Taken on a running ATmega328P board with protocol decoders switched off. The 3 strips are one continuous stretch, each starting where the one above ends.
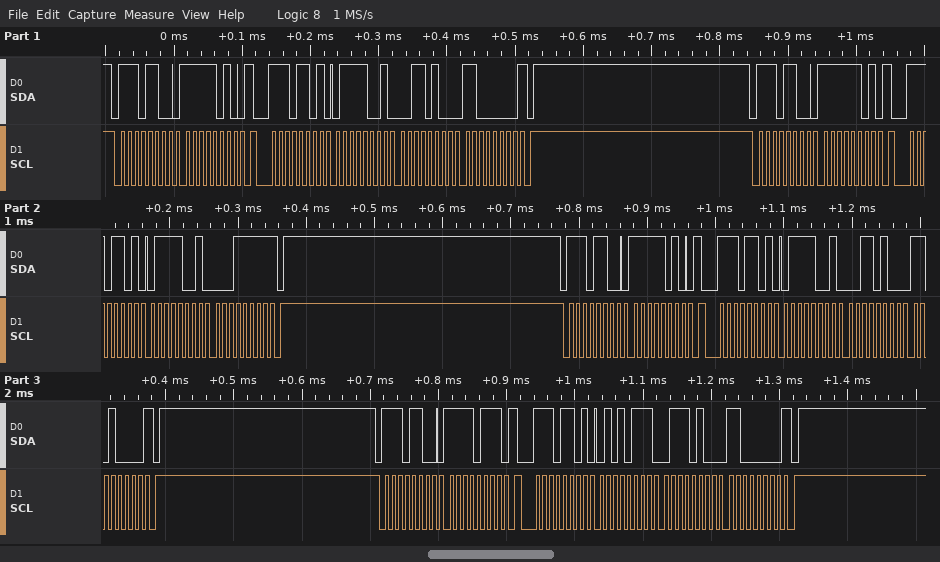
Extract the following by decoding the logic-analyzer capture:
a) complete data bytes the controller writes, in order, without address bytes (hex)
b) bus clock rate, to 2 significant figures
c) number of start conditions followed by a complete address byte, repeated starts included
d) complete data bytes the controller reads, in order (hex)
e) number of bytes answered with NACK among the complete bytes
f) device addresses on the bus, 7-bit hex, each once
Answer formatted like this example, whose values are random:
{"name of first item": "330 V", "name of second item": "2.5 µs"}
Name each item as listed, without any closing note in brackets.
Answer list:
{"complete data bytes the controller writes, in order, without address bytes": "FA FD FA F7", "bus clock rate, to 2 significant figures": "100 kHz", "number of start conditions followed by a complete address byte, repeated starts included": "8", "complete data bytes the controller reads, in order": "79 34 C0 79 1F 79 34 D0 57 74 C0", "number of bytes answered with NACK among the complete bytes": "4", "device addresses on the bus, 7-bit hex, each once": "0x76"}
